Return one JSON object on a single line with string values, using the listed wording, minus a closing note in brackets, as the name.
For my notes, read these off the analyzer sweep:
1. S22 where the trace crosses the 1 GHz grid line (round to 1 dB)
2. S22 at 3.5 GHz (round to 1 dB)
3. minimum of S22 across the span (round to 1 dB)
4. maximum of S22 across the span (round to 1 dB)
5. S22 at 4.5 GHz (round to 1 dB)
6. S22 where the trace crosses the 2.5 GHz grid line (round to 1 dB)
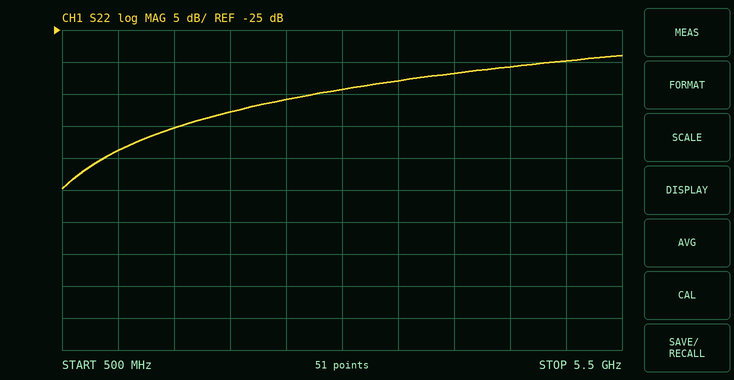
{"S22 where the trace crosses the 1 GHz grid line": "-44 dB", "S22 at 3.5 GHz": "-33 dB", "minimum of S22 across the span": "-50 dB", "maximum of S22 across the span": "-29 dB", "S22 at 4.5 GHz": "-31 dB", "S22 where the trace crosses the 2.5 GHz grid line": "-36 dB"}
